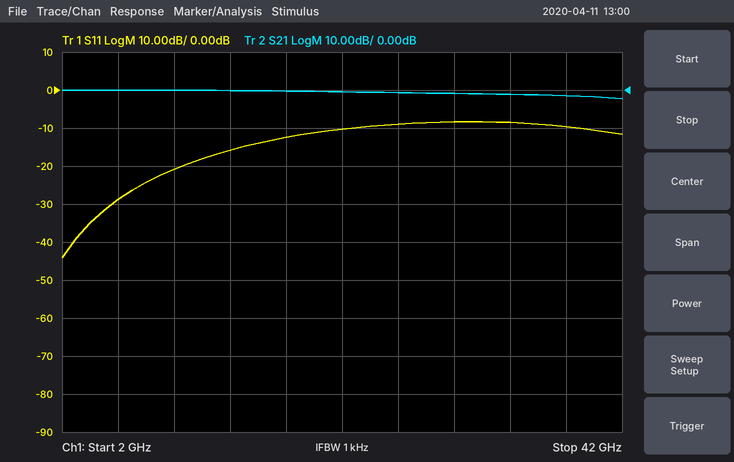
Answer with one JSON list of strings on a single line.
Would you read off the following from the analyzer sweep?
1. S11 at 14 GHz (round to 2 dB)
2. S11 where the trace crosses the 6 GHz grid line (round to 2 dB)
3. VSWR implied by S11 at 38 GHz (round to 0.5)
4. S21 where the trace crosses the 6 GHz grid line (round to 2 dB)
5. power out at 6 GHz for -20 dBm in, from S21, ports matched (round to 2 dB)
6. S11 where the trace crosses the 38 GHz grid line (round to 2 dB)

["-16 dB", "-28 dB", "2.0", "0 dB", "-20 dBm", "-10 dB"]
